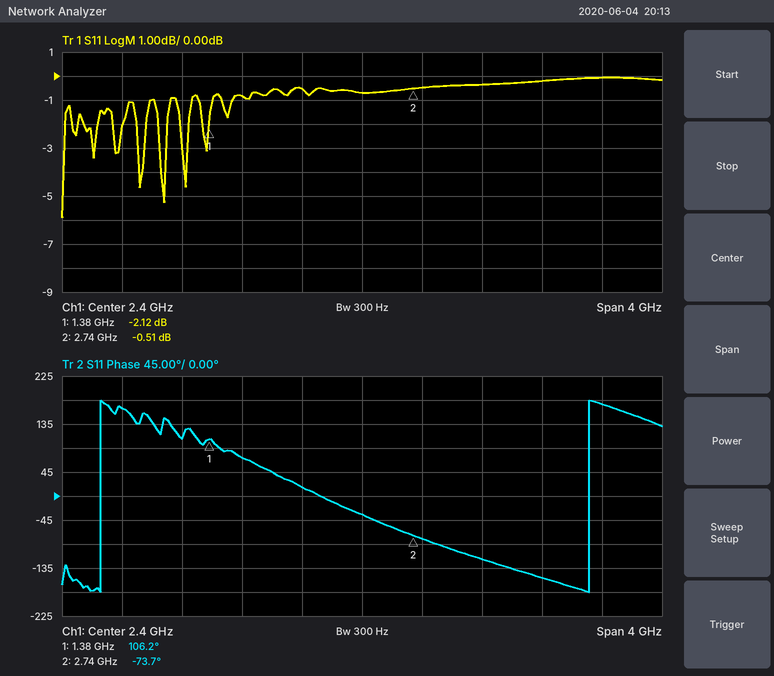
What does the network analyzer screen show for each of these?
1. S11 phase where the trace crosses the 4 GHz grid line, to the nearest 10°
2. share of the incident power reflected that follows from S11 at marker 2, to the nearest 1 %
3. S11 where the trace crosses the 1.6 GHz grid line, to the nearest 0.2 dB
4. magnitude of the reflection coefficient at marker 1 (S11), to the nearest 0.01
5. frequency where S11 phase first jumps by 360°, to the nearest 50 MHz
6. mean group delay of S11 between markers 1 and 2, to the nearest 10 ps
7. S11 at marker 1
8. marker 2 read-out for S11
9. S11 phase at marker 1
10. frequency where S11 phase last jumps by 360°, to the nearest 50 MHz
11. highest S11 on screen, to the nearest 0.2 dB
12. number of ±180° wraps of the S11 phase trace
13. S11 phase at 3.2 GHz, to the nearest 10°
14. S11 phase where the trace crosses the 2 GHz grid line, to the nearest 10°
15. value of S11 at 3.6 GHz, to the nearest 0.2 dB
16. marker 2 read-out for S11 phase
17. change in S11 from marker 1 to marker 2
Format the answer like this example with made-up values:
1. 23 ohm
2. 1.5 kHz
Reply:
1. 170°
2. 89 %
3. -0.8 dB
4. 0.78
5. 650 MHz
6. 370 ps
7. -2.12 dB
8. -0.51 dB
9. 106.2°
10. 3.90 GHz
11. 0.0 dB
12. 2
13. -120°
14. 20°
15. -0.2 dB
16. -73.7°
17. 1.61 dB
